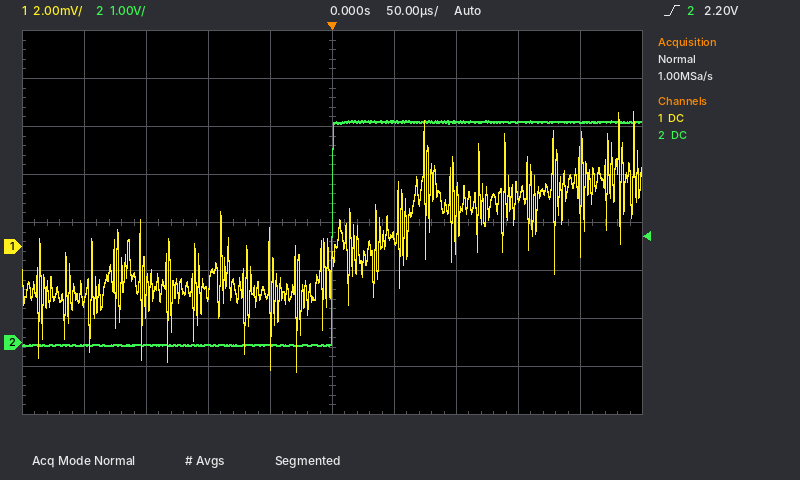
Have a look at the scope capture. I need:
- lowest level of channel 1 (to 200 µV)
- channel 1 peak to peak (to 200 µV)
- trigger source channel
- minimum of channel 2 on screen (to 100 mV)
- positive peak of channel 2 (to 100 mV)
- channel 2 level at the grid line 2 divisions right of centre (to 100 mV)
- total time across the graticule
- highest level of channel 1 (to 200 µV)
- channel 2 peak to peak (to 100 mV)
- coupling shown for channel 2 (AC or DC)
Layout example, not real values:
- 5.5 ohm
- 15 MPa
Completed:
- -5.2 mV
- 10.8 mV
- channel 2
- -100 mV
- 4.6 V
- 4.6 V
- 500 µs
- 5.6 mV
- 4.7 V
- DC
